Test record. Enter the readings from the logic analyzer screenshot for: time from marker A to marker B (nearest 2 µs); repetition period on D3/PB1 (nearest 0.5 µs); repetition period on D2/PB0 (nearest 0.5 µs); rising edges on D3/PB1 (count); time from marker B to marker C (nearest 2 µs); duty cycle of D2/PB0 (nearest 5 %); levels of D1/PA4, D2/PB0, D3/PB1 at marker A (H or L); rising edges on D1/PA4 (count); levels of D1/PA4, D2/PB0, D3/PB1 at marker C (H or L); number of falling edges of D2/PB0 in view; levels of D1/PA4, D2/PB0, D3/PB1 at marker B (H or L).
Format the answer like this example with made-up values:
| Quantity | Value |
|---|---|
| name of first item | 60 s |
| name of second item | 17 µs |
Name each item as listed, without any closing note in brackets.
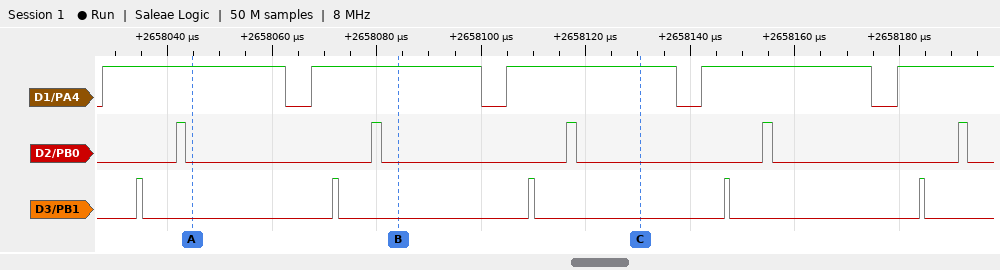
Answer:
| Quantity | Value |
|---|---|
| time from marker A to marker B | 40 µs |
| repetition period on D3/PB1 | 37.5 µs |
| repetition period on D2/PB0 | 37.5 µs |
| rising edges on D3/PB1 | 5 |
| time from marker B to marker C | 46 µs |
| duty cycle of D2/PB0 | 5 % |
| levels of D1/PA4, D2/PB0, D3/PB1 at marker A | D1/PA4=H, D2/PB0=L, D3/PB1=L |
| rising edges on D1/PA4 | 5 |
| levels of D1/PA4, D2/PB0, D3/PB1 at marker C | D1/PA4=H, D2/PB0=L, D3/PB1=L |
| number of falling edges of D2/PB0 in view | 5 |
| levels of D1/PA4, D2/PB0, D3/PB1 at marker B | D1/PA4=H, D2/PB0=L, D3/PB1=L |
